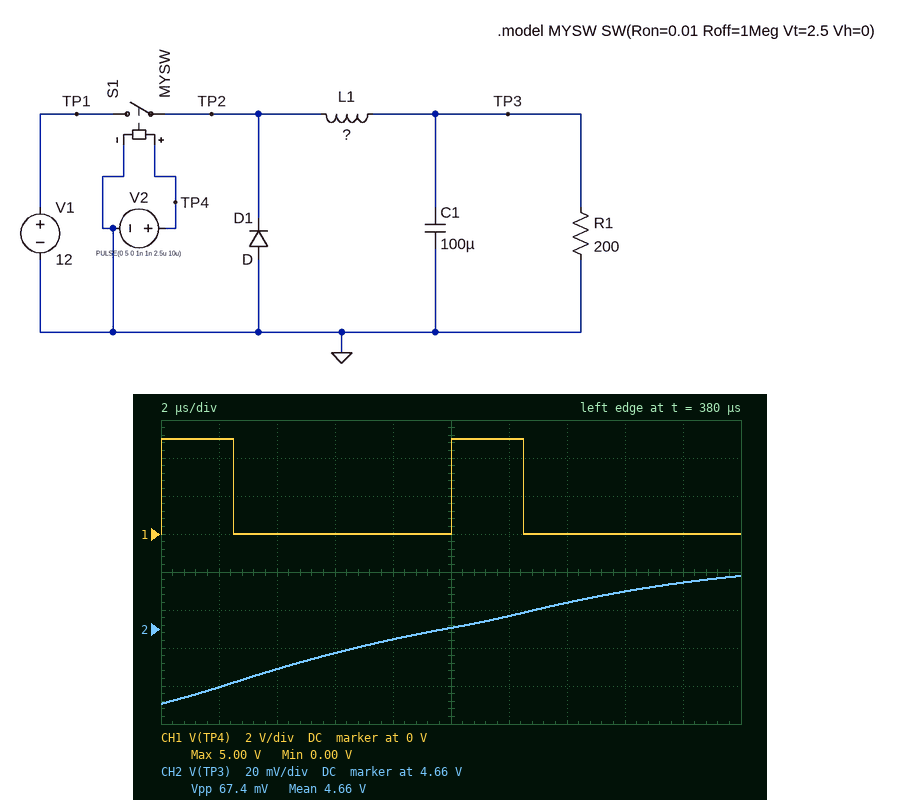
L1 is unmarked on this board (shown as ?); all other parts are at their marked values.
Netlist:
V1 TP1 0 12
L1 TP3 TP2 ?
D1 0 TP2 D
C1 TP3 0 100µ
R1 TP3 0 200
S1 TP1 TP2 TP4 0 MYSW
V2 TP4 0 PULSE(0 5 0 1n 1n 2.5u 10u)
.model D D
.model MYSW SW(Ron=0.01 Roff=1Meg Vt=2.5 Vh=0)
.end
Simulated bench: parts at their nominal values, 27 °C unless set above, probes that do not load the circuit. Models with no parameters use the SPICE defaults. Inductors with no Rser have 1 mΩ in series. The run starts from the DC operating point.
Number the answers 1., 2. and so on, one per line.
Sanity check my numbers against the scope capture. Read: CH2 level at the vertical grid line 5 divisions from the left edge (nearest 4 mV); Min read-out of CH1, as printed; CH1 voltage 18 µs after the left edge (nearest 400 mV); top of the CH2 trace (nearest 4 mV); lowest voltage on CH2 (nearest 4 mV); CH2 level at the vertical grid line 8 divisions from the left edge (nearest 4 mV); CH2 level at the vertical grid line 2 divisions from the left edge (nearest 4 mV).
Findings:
1. 4.660 V
2. 0.00 V
3. 0 V
4. 4.688 V
5. 4.620 V
6. 4.680 V
7. 4.640 V
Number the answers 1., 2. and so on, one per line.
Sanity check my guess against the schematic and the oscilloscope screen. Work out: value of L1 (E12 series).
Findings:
1. 180 µH
